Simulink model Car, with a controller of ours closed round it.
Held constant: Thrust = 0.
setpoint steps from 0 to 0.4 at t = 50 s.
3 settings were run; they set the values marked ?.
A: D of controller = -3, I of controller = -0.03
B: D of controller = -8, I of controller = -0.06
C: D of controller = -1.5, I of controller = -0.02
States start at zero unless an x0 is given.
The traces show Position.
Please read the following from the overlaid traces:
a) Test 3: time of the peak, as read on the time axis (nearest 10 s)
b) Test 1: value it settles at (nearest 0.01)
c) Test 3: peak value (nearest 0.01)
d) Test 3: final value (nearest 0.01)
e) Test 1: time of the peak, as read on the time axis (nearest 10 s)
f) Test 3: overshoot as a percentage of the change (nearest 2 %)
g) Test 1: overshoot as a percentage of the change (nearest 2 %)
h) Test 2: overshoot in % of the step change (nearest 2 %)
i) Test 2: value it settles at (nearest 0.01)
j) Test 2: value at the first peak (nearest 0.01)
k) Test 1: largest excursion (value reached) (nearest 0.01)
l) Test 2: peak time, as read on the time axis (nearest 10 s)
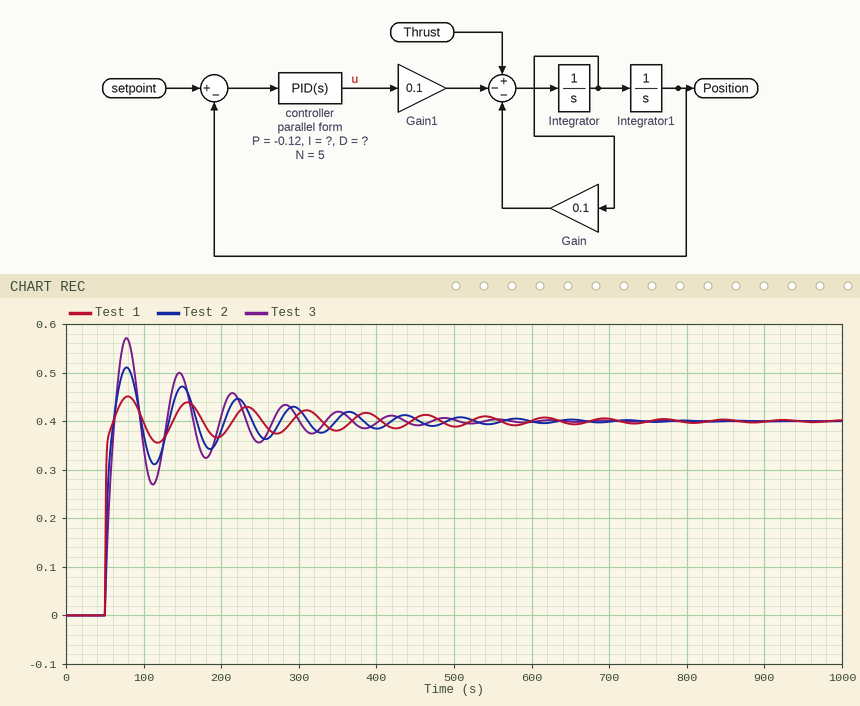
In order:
80 s
0.40
0.57
0.40
80 s
42 %
12 %
28 %
0.40
0.51
0.45
80 s
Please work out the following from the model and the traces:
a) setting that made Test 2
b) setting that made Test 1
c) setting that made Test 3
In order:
A
B
C
